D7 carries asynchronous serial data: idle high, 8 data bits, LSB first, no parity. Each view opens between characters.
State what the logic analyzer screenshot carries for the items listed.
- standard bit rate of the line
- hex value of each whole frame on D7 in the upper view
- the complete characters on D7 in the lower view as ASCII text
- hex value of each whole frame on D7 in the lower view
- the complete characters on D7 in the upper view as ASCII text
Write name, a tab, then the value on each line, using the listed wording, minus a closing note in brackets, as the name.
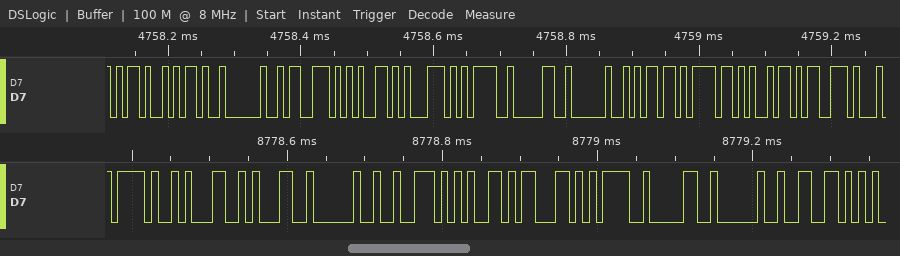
standard bit rate of the line	115200 baud
hex value of each whole frame on D7 in the upper view	2D, 2D, 20, 73, 65, 71, 3D, 30, 20, 6D, 6F, 69, 73
the complete characters on D7 in the lower view as ASCII text	"/11 rec=0 f"
hex value of each whole frame on D7 in the lower view	2F, 31, 31, 20, 72, 65, 63, 3D, 30, 20, 66
the complete characters on D7 in the upper view as ASCII text	"-- seq=0 mois"
